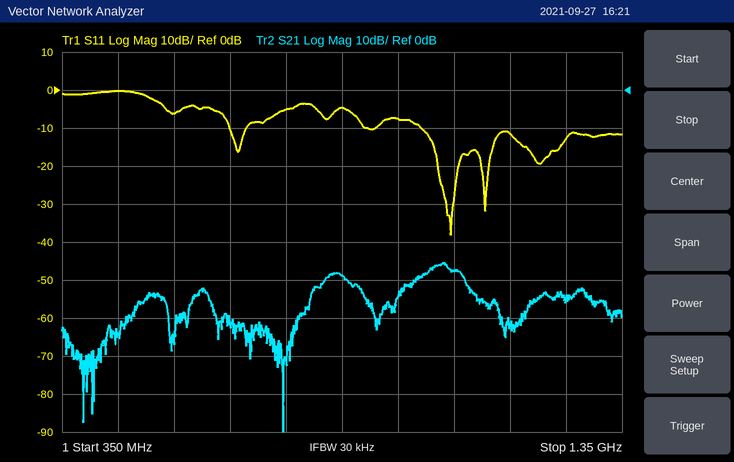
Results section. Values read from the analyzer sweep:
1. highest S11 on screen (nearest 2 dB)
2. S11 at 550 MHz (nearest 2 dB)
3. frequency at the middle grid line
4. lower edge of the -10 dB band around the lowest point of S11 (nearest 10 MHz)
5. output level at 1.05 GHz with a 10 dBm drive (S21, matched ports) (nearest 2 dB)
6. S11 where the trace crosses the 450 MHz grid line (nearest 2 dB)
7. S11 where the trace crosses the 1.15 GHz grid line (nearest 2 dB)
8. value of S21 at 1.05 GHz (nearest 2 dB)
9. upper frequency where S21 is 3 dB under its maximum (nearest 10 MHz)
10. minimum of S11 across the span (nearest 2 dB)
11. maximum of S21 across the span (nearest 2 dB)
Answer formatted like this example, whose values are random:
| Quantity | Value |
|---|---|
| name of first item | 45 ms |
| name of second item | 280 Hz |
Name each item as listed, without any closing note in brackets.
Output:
| Quantity | Value |
|---|---|
| highest S11 on screen | 0 dB |
| S11 at 550 MHz | -6 dB |
| frequency at the middle grid line | 850 MHz |
| lower edge of the -10 dB band around the lowest point of S11 | 990 MHz |
| output level at 1.05 GHz with a 10 dBm drive (S21, matched ports) | -38 dBm |
| S11 where the trace crosses the 450 MHz grid line | 0 dB |
| S11 where the trace crosses the 1.15 GHz grid line | -12 dB |
| value of S21 at 1.05 GHz | -48 dB |
| upper frequency where S21 is 3 dB under its maximum | 1.06 GHz |
| minimum of S11 across the span | -38 dB |
| maximum of S21 across the span | -46 dB |
